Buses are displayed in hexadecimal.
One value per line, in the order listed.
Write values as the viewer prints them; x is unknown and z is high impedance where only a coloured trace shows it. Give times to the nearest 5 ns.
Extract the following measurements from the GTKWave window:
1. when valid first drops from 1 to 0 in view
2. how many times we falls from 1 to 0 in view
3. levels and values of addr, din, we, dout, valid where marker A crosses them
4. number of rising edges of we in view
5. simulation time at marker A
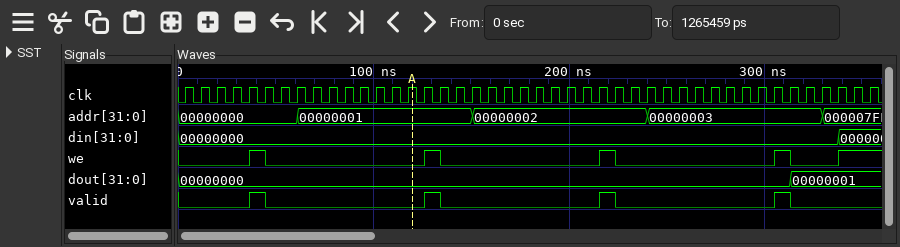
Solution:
45 ns
4
addr=00000001, din=00000000, we=0, dout=00000000, valid=0
5
120 ns
